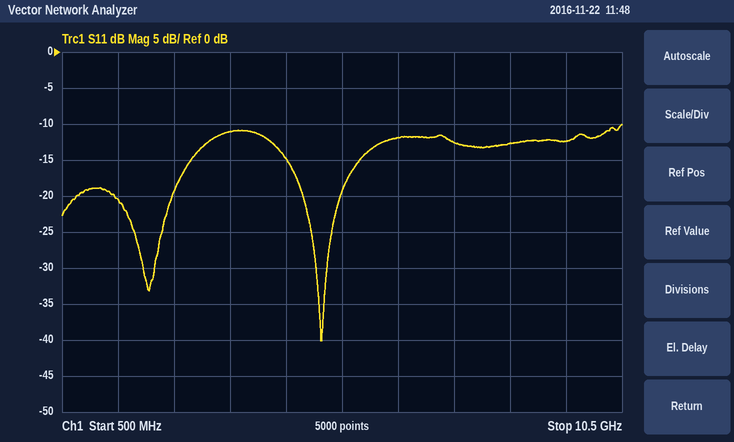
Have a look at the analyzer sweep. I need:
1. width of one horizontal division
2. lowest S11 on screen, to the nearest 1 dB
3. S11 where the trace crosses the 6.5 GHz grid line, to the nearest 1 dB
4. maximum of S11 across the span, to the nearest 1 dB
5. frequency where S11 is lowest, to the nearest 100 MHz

1 GHz
-40 dB
-12 dB
-10 dB
5.1 GHz
